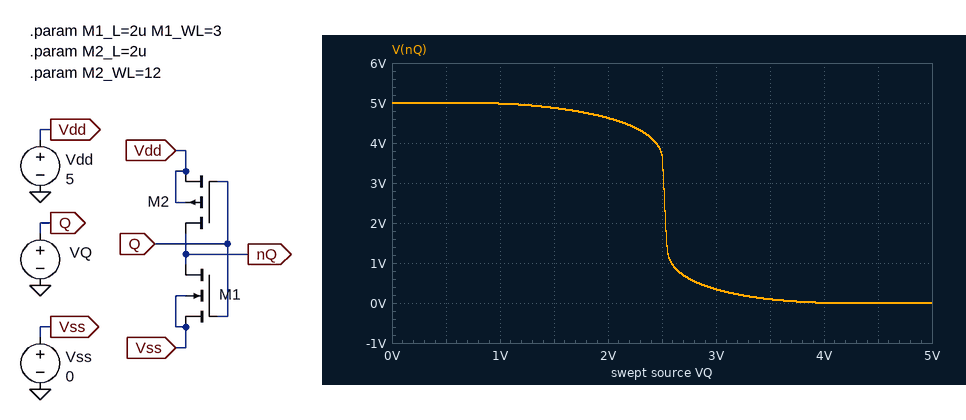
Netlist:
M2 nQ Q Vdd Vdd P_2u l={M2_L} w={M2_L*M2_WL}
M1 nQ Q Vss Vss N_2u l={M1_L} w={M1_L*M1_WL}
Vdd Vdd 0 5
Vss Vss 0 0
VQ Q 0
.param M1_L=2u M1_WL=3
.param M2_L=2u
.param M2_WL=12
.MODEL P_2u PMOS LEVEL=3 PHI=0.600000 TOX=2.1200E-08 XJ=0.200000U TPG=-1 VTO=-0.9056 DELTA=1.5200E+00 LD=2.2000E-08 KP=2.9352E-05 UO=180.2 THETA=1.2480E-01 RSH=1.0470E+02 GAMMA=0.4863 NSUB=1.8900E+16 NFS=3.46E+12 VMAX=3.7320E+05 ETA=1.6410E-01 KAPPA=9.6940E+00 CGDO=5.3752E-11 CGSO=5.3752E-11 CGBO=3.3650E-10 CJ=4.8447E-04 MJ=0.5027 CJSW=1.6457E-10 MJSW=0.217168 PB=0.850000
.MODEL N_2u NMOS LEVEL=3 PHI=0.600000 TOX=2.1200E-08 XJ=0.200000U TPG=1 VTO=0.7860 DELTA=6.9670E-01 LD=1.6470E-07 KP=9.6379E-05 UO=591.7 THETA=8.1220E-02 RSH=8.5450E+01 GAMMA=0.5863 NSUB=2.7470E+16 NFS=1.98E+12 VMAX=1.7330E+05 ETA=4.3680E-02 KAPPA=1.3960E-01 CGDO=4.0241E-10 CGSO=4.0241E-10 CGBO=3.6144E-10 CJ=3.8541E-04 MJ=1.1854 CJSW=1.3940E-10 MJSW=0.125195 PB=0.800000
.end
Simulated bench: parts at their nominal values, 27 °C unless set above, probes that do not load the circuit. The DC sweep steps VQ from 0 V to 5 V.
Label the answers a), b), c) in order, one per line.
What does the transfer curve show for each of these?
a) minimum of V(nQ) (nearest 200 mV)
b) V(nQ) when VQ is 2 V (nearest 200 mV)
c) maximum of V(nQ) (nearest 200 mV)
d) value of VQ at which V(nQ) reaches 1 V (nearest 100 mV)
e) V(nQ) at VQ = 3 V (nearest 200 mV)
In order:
a) 0 V
b) 4.6 V
c) 5.0 V
d) 2.6 V
e) 400 mV
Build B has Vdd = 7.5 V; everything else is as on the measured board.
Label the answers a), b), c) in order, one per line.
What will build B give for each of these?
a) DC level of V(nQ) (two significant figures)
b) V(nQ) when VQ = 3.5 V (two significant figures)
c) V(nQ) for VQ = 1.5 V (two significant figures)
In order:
a) 7.5 V
b) 6.2 V
c) 7.4 V
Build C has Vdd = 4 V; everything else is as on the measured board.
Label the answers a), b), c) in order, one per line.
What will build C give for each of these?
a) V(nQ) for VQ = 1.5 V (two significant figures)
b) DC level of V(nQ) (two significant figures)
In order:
a) 3.8 V
b) 4.0 V
